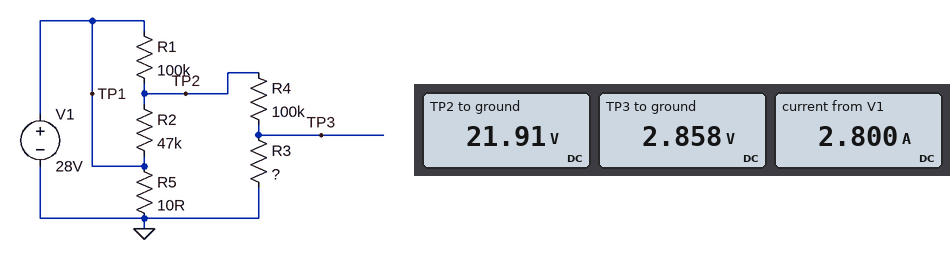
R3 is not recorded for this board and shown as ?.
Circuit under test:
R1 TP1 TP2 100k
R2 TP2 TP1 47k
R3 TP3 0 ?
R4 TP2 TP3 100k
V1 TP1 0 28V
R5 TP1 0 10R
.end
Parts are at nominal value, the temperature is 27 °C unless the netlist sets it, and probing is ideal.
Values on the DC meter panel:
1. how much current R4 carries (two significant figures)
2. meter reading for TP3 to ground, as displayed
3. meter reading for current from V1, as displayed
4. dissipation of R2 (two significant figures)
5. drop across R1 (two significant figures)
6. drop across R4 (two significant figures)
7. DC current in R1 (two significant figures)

190 µA
2.858 V
2.800 A
790 µW
6.1 V
19 V
61 µA
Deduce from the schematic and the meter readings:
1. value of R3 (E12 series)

15 kΩ
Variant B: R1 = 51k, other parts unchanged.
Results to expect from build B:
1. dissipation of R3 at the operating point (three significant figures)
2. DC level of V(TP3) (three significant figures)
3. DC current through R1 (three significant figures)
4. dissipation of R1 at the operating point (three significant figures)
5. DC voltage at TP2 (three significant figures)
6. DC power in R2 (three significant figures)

605 µW
3.01 V
96.3 µA
473 µW
23.1 V
513 µW
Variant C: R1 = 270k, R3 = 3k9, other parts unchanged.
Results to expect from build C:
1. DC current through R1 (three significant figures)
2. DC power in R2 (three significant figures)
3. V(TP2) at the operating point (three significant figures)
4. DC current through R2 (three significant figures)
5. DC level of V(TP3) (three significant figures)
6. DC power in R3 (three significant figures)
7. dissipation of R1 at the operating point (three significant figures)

28.8 µA
1.29 mW
20.2 V
166 µA
759 mV
148 µW
225 µW
